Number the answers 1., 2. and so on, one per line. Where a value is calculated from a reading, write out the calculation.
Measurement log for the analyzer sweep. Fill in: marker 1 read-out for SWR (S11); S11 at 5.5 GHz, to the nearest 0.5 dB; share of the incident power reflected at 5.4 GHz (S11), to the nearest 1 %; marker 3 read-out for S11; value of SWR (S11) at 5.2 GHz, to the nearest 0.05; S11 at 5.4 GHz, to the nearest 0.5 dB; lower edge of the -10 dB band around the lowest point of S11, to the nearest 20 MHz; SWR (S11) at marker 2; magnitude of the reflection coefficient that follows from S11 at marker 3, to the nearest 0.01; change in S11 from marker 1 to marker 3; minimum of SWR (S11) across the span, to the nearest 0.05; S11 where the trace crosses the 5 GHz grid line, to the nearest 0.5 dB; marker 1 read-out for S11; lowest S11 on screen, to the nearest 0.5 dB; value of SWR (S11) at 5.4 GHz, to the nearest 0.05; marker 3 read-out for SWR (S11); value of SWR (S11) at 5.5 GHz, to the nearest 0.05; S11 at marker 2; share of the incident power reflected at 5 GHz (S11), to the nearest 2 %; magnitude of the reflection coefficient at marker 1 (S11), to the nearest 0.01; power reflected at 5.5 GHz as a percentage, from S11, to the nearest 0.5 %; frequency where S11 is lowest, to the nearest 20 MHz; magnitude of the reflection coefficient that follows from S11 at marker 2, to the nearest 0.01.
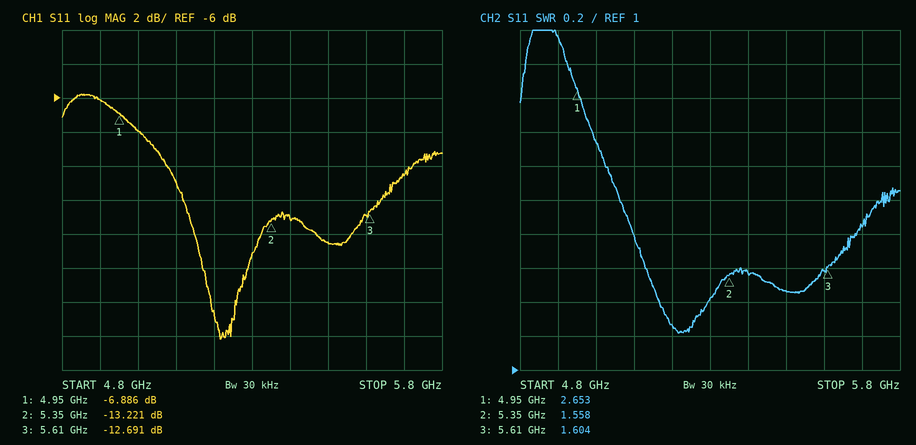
1. 2.653
2. -14.5 dB
3. 10^(-13/10) ≈ 5 %
4. -12.691 dB
5. 1.25
6. -13.0 dB
7. 5.08 GHz
8. 1.558
9. 10^(-12.691/20) ≈ 0.23
10. -12.691 − (-6.886) = -5.805 dB
11. 1.20
12. -8.0 dB
13. -6.886 dB
14. -20.0 dB
15. 1.55
16. 1.604
17. 1.45
18. -13.221 dB
19. 10^(-8/10) ≈ 16 %
20. 10^(-6.886/20) ≈ 0.45
21. 10^(-14.5/10) ≈ 3.5 %
22. 5.22 GHz
23. 10^(-13.221/20) ≈ 0.22
